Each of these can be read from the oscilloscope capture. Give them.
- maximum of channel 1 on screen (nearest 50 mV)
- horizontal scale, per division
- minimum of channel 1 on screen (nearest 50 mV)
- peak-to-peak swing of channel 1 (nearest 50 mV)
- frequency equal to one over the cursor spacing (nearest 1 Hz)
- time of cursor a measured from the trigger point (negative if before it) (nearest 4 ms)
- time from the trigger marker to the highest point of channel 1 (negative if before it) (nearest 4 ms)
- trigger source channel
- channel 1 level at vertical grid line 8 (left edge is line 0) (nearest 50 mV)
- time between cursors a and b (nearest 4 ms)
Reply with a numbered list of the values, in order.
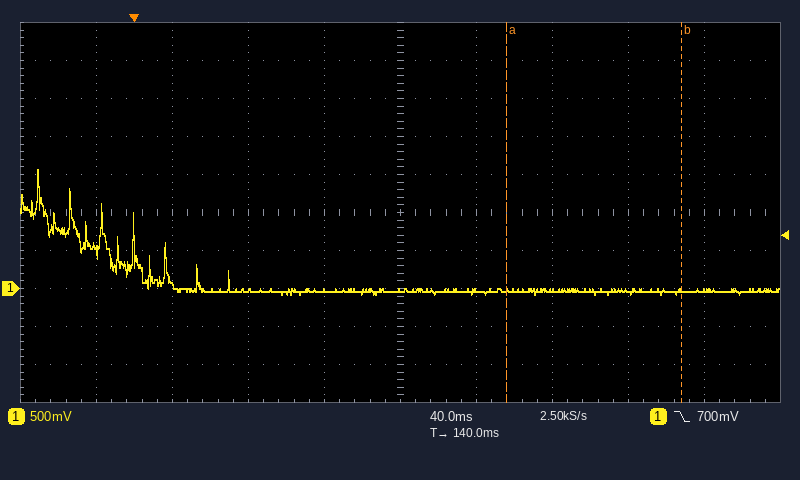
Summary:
1. 1.55 V
2. 40 ms
3. -100 mV
4. 1.65 V
5. 11 Hz
6. +196 ms
7. -52 ms
8. channel 1
9. -50 mV
10. 92 ms
